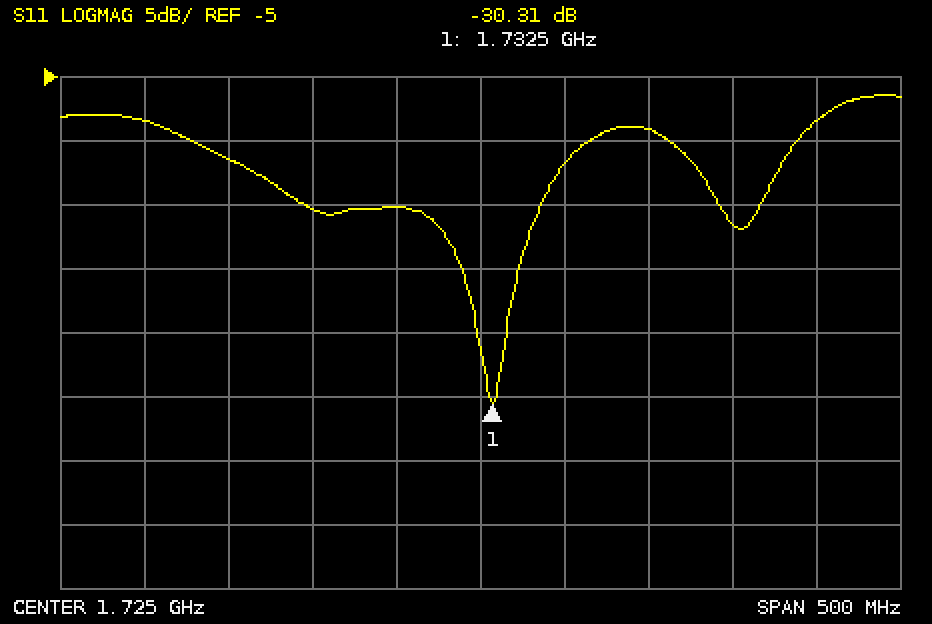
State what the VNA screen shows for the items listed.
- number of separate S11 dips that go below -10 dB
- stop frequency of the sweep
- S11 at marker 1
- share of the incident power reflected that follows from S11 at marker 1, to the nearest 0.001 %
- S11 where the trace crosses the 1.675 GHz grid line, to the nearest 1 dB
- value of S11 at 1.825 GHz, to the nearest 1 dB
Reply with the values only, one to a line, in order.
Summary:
2
1.975 GHz
-30.31 dB
0.093 %
-15 dB
-9 dB
